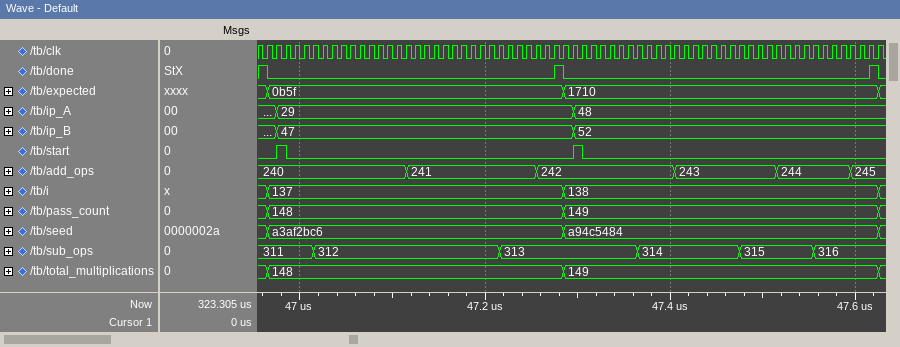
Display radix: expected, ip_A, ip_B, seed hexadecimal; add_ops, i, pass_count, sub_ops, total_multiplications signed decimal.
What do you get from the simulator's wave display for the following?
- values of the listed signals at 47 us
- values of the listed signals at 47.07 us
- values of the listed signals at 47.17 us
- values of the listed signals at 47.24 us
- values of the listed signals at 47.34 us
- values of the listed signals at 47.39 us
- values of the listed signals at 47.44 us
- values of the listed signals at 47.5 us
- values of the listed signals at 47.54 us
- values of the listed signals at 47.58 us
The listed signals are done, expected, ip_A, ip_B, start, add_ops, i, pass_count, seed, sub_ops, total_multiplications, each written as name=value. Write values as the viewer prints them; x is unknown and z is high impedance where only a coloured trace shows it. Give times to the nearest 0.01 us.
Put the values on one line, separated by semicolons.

done=0, expected=0b5f, ip_A=29, ip_B=47, start=0, add_ops=240, i=137, pass_count=148, seed=a3af2bc6, sub_ops=311, total_multiplications=148; done=0, expected=0b5f, ip_A=29, ip_B=47, start=0, add_ops=240, i=137, pass_count=148, seed=a3af2bc6, sub_ops=312, total_multiplications=148; done=0, expected=0b5f, ip_A=29, ip_B=47, start=0, add_ops=241, i=137, pass_count=148, seed=a3af2bc6, sub_ops=312, total_multiplications=148; done=0, expected=0b5f, ip_A=29, ip_B=47, start=0, add_ops=241, i=137, pass_count=148, seed=a3af2bc6, sub_ops=313, total_multiplications=148; done=0, expected=1710, ip_A=48, ip_B=52, start=0, add_ops=242, i=138, pass_count=149, seed=a94c5484, sub_ops=313, total_multiplications=149; done=0, expected=1710, ip_A=48, ip_B=52, start=0, add_ops=242, i=138, pass_count=149, seed=a94c5484, sub_ops=314, total_multiplications=149; done=0, expected=1710, ip_A=48, ip_B=52, start=0, add_ops=243, i=138, pass_count=149, seed=a94c5484, sub_ops=314, total_multiplications=149; done=0, expected=1710, ip_A=48, ip_B=52, start=0, add_ops=243, i=138, pass_count=149, seed=a94c5484, sub_ops=315, total_multiplications=149; done=0, expected=1710, ip_A=48, ip_B=52, start=0, add_ops=244, i=138, pass_count=149, seed=a94c5484, sub_ops=315, total_multiplications=149; done=0, expected=1710, ip_A=48, ip_B=52, start=0, add_ops=244, i=138, pass_count=149, seed=a94c5484, sub_ops=316, total_multiplications=149
